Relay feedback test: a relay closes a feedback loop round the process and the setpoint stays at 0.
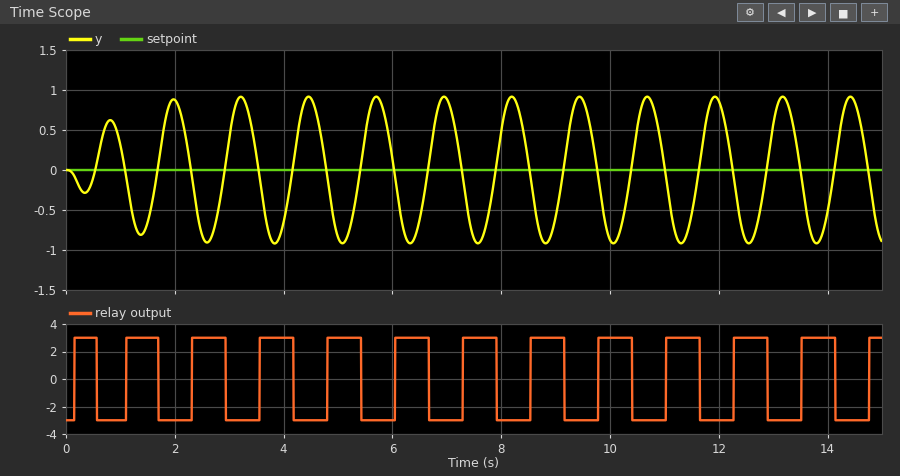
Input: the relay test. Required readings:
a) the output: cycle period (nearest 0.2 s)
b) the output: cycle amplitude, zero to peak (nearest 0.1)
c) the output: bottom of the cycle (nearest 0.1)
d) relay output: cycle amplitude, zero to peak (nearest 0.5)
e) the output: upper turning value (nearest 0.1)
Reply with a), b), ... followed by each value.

a) 1.2 s
b) 0.9
c) -0.9
d) 3.0
e) 0.9
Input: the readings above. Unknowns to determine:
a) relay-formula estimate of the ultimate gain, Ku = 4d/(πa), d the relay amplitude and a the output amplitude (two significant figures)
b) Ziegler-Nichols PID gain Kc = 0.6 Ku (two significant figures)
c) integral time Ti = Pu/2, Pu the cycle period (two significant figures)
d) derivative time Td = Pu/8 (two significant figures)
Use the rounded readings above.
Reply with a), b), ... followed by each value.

a) 4.2
b) 2.5
c) 0.60 s
d) 0.15 s
